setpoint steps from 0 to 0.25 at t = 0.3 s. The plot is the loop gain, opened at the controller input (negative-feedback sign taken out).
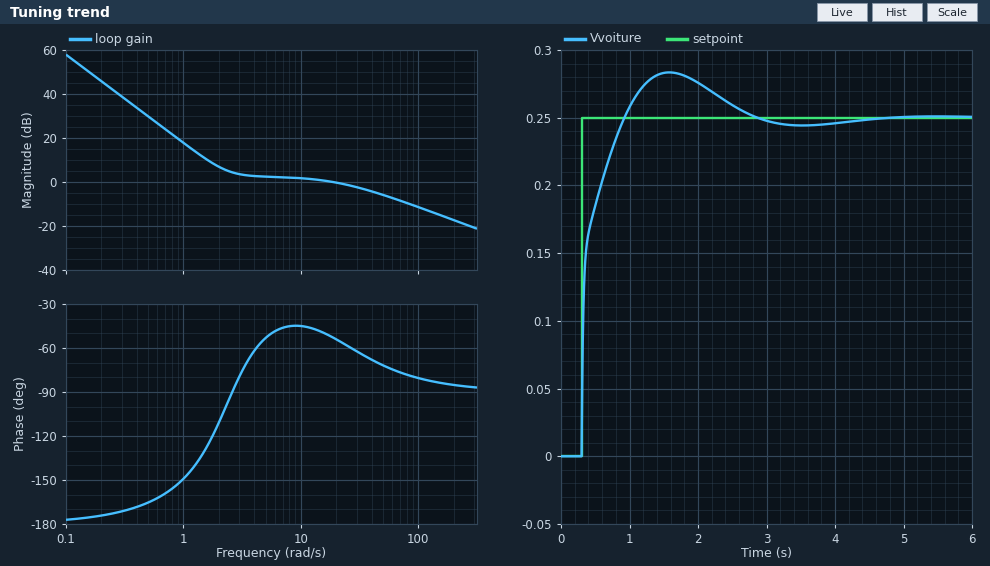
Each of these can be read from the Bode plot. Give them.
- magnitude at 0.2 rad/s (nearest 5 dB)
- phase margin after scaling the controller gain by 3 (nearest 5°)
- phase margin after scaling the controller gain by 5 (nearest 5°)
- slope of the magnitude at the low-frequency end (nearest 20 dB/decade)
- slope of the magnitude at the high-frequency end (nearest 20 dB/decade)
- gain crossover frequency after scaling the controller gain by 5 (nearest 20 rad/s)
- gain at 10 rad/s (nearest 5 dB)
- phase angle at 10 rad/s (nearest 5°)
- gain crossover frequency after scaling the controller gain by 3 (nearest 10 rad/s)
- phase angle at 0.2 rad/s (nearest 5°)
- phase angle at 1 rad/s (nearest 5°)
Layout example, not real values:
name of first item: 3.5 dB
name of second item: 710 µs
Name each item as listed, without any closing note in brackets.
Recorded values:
magnitude at 0.2 rad/s: 45 dB
phase margin after scaling the controller gain by 3: 100°
phase margin after scaling the controller gain by 5: 95°
slope of the magnitude at the low-frequency end: -40 dB/decade
slope of the magnitude at the high-frequency end: -20 dB/decade
gain crossover frequency after scaling the controller gain by 5: 140 rad/s
gain at 10 rad/s: 0 dB
phase angle at 10 rad/s: -45°
gain crossover frequency after scaling the controller gain by 3: 80 rad/s
phase angle at 0.2 rad/s: -175°
phase angle at 1 rad/s: -150°
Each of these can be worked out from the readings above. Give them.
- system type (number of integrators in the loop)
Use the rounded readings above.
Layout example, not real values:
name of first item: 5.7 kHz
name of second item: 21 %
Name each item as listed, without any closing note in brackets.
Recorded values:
system type: 2
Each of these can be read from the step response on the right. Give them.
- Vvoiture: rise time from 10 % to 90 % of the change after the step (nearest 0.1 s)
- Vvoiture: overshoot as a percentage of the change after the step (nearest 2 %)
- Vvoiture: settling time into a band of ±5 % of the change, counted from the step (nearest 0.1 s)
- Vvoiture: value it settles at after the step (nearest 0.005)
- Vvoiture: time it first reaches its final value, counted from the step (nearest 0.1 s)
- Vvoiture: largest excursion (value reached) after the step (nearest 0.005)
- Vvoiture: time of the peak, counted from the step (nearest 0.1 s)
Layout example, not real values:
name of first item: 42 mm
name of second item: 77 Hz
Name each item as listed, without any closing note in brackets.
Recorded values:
Vvoiture: rise time from 10 % to 90 % of the change after the step: 0.4 s
Vvoiture: overshoot as a percentage of the change after the step: 14 %
Vvoiture: settling time into a band of ±5 % of the change, counted from the step: 2.1 s
Vvoiture: value it settles at after the step: 0.250
Vvoiture: time it first reaches its final value, counted from the step: 0.6 s
Vvoiture: largest excursion (value reached) after the step: 0.285
Vvoiture: time of the peak, counted from the step: 1.3 s
